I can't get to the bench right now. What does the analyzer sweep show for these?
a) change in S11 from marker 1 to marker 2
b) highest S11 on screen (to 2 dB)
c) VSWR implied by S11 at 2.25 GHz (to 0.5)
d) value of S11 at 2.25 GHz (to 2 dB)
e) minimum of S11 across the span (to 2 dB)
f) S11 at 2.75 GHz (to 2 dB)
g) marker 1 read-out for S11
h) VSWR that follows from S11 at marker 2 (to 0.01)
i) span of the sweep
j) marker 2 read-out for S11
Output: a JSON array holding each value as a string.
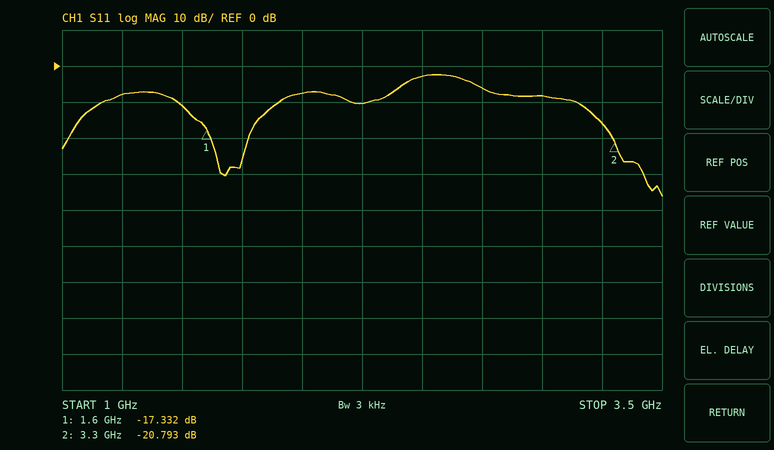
["-3.461 dB", "-2 dB", "2.0", "-10 dB", "-36 dB", "-6 dB", "-17.332 dB", "1.20", "2.5 GHz", "-20.793 dB"]
